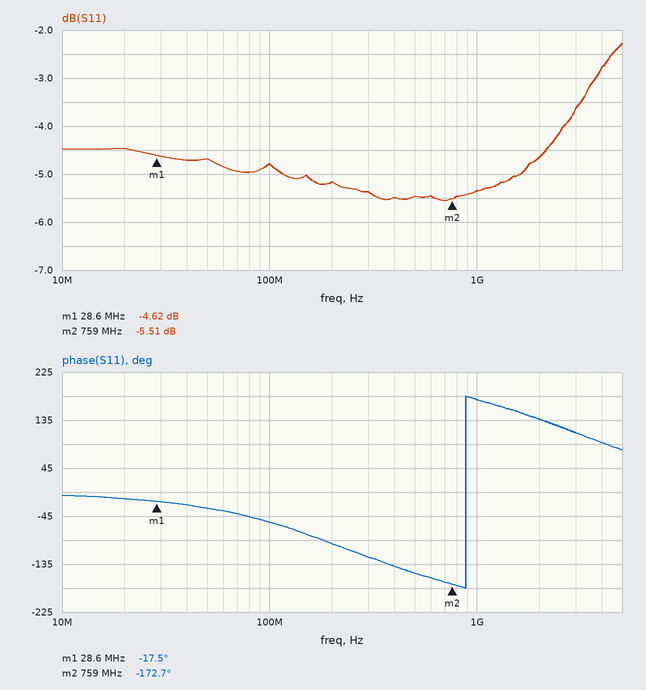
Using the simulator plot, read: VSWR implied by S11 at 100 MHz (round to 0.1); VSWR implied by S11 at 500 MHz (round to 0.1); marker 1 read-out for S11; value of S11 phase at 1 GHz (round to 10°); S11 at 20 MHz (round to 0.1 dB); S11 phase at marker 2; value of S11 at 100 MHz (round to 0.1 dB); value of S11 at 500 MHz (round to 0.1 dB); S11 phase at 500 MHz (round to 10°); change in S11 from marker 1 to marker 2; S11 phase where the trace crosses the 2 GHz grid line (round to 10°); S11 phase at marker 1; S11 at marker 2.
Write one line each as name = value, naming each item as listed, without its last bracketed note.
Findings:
VSWR implied by S11 at 100 MHz = 3.7
VSWR implied by S11 at 500 MHz = 3.3
marker 1 read-out for S11 = -4.62 dB
value of S11 phase at 1 GHz = 170°
S11 at 20 MHz = -4.5 dB
S11 phase at marker 2 = -172.7°
value of S11 at 100 MHz = -4.8 dB
value of S11 at 500 MHz = -5.5 dB
S11 phase at 500 MHz = -150°
change in S11 from marker 1 to marker 2 = -0.89 dB
S11 phase where the trace crosses the 2 GHz grid line = 140°
S11 phase at marker 1 = -17.5°
S11 at marker 2 = -5.51 dB
